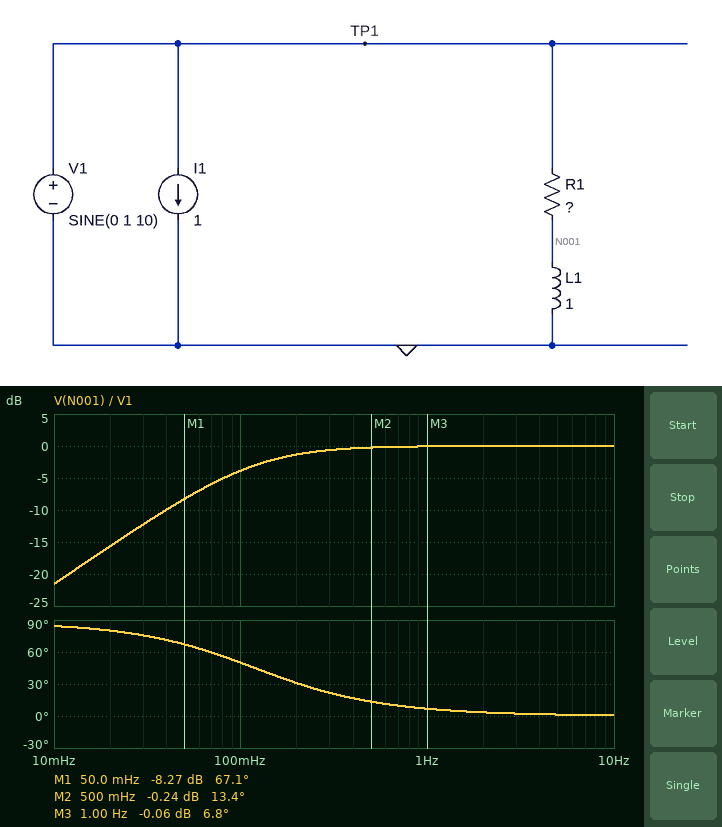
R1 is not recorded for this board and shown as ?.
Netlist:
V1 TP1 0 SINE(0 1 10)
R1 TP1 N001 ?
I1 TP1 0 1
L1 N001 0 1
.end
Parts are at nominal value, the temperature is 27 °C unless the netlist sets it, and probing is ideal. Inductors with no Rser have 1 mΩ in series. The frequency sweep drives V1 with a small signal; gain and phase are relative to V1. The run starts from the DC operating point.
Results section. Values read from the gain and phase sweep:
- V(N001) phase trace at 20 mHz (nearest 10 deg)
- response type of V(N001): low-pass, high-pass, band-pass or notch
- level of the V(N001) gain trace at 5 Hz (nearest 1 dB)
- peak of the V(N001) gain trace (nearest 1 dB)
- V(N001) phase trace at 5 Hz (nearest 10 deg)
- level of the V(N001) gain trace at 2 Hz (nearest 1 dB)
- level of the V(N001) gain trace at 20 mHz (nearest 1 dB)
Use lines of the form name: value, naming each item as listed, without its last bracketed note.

V(N001) phase trace at 20 mHz: 80 deg
response type of V(N001): low-pass, high-pass, band-pass or notch: high-pass
level of the V(N001) gain trace at 5 Hz: 0 dB
peak of the V(N001) gain trace: 0 dB
V(N001) phase trace at 5 Hz: 0 deg
level of the V(N001) gain trace at 2 Hz: 0 dB
level of the V(N001) gain trace at 20 mHz: -16 dB
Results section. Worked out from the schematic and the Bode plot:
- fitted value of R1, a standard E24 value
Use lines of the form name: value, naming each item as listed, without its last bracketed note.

fitted value of R1, a standard E24 value: 0.75 Ω
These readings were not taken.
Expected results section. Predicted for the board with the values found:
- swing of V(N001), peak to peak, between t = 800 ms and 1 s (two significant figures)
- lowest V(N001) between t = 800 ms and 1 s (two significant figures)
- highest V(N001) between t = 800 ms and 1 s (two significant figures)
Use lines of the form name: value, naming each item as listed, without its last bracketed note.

swing of V(N001), peak to peak, between t = 800 ms and 1 s: 2.0 V
lowest V(N001) between t = 800 ms and 1 s: -1.0 V
highest V(N001) between t = 800 ms and 1 s: 990 mV
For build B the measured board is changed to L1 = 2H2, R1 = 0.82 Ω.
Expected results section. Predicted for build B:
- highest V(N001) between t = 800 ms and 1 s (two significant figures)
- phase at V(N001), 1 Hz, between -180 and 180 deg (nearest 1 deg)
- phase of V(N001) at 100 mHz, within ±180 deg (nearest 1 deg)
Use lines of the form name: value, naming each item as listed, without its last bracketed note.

highest V(N001) between t = 800 ms and 1 s: 1.0 V
phase at V(N001), 1 Hz, between -180 and 180 deg: 3 deg
phase of V(N001) at 100 mHz, within ±180 deg: 31 deg
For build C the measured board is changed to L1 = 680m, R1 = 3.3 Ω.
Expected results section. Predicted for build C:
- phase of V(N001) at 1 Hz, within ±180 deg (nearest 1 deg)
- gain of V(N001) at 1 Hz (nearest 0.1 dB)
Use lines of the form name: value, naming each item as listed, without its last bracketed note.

phase of V(N001) at 1 Hz, within ±180 deg: 38 deg
gain of V(N001) at 1 Hz: -2.0 dB
